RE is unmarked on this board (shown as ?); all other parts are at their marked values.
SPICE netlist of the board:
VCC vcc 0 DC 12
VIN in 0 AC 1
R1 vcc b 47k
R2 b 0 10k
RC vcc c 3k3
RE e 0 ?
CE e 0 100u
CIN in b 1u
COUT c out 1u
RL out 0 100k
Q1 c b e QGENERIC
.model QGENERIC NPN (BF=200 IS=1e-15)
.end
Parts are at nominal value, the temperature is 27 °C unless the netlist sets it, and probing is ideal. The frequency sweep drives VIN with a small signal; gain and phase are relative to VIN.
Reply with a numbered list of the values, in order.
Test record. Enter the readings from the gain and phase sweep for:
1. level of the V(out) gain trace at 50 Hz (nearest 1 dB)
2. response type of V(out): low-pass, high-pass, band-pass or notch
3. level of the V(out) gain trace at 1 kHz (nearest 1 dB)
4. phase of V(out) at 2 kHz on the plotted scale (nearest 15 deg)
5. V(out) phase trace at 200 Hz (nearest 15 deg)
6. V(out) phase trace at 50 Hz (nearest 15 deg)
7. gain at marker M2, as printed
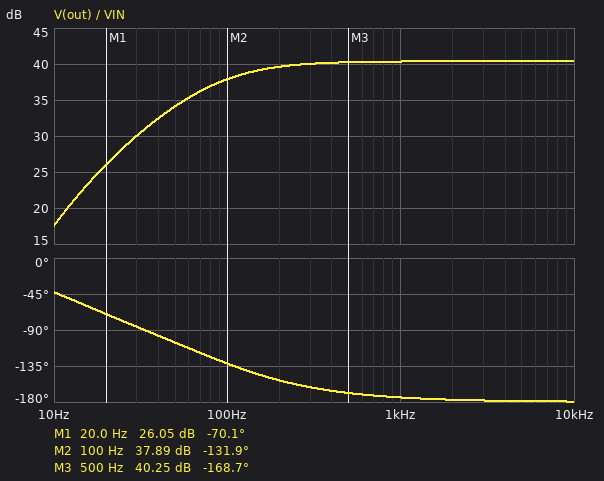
1. 34 dB
2. high-pass
3. 40 dB
4. -180 deg
5. -150 deg
6. -105 deg
7. 37.89 dB
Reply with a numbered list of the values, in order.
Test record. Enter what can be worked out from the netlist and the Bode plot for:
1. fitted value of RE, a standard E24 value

1. 1.6 kΩ
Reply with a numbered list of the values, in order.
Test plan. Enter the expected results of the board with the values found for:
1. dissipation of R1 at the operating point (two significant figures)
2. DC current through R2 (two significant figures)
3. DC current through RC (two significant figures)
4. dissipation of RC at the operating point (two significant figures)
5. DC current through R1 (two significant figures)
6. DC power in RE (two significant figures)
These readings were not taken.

1. 2.1 mW
2. 210 µA
3. 850 µA
4. 2.4 mW
5. 210 µA
6. 1.2 mW
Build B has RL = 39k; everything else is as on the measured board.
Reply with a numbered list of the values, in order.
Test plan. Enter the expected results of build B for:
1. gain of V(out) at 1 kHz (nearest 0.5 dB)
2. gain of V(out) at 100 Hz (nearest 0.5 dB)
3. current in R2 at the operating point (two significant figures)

1. 40.0 dB
2. 37.5 dB
3. 210 µA
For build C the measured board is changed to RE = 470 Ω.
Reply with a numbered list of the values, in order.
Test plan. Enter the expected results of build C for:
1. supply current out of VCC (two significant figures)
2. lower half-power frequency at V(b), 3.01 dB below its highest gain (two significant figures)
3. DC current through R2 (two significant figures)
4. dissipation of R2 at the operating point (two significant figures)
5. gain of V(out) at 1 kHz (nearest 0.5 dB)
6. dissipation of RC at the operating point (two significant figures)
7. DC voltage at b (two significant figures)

1. 2.9 mA
2. 100 Hz
3. 200 µA
4. 400 µW
5. 50.0 dB
6. 23 mW
7. 2.0 V
